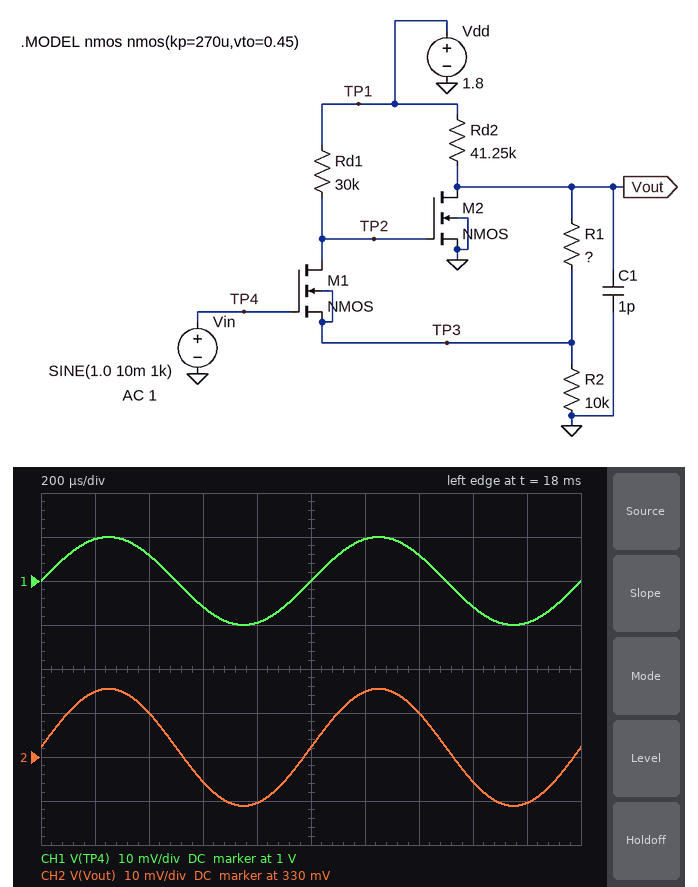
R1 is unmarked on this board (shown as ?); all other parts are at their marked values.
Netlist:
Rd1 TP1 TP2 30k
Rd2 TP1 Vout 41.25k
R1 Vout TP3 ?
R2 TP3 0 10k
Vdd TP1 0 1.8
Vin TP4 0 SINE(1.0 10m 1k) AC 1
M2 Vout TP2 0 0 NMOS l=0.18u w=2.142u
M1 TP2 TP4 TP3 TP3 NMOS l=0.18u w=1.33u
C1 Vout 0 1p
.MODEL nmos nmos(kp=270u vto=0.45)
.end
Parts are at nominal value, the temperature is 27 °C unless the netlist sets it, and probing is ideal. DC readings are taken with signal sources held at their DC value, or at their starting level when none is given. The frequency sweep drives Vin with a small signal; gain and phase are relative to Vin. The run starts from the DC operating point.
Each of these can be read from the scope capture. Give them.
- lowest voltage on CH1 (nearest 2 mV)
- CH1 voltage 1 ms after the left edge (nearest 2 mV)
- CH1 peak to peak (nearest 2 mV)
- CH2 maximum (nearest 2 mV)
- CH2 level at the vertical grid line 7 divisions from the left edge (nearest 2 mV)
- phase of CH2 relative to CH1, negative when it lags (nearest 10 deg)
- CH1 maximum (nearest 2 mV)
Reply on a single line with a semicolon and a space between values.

990 mV; 1.000 V; 20 mV; 346 mV; 340 mV; 0 deg; 1.010 V
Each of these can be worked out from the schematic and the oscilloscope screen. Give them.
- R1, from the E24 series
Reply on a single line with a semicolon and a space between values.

3.9 kΩ
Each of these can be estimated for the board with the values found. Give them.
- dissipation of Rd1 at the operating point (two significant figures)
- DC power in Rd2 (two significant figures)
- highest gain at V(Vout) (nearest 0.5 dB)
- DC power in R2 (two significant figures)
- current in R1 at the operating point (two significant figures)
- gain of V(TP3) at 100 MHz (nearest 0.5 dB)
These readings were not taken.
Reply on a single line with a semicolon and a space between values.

47 µW; 52 µW; 2.5 dB; 12 µW; 4.7 µA; -0.5 dB
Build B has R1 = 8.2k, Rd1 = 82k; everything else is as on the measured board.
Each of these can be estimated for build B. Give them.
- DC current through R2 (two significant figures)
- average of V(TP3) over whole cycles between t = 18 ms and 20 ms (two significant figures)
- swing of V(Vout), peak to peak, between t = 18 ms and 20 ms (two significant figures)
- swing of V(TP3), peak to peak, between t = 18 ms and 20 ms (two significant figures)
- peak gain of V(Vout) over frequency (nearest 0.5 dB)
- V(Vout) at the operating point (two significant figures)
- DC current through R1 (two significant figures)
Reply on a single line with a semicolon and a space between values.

41 µA; 410 mV; 15 mV; 8.7 mV; -2.5 dB; 620 mV; 25 µA
